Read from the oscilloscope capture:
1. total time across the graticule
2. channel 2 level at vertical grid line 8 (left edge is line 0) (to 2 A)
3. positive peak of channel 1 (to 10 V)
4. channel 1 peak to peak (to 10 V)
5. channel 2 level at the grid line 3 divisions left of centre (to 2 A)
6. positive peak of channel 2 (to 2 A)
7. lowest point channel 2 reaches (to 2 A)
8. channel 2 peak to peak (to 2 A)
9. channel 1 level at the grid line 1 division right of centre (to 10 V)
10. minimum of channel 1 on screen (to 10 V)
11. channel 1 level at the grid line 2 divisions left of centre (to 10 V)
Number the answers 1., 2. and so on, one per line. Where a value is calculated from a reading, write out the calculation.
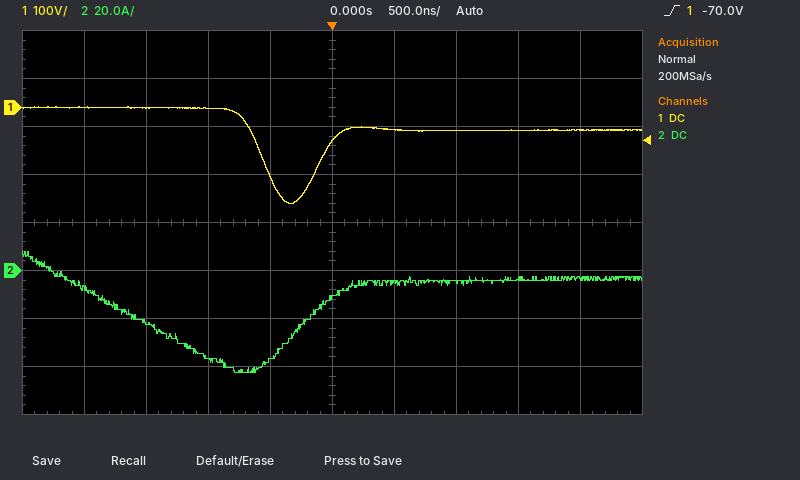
1. 5 µs
2. -4 A
3. 0 V
4. 0 V − (-200 V) = 200 V
5. -22 A
6. 8 A
7. -42 A
8. 8 A − (-42 A) = 50 A
9. -50 V
10. -200 V
11. 0 V
